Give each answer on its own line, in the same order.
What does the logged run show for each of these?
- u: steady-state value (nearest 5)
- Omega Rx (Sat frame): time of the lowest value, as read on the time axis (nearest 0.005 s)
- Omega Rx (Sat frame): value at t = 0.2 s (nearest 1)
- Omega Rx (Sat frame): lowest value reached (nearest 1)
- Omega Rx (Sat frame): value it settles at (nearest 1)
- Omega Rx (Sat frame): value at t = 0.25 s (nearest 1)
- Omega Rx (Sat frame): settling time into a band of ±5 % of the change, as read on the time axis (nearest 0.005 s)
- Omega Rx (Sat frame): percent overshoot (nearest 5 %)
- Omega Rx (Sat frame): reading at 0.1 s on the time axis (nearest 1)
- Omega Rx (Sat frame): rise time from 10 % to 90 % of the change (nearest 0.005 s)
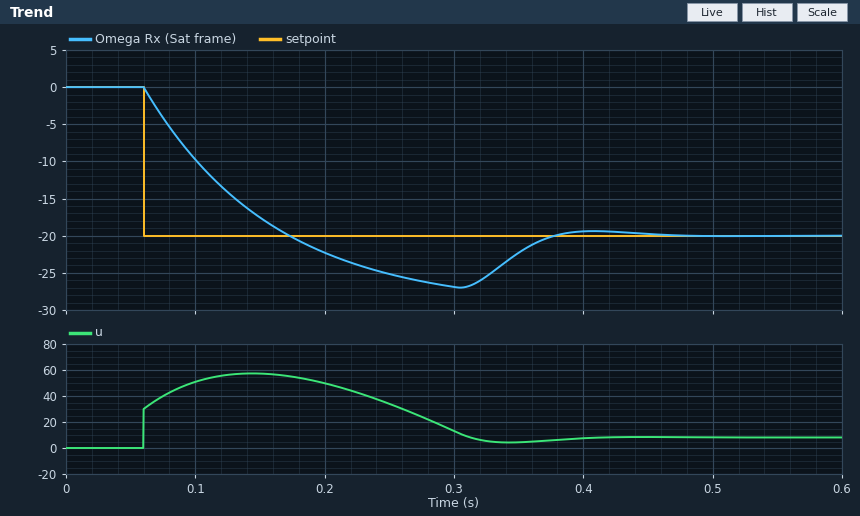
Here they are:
10
0.305 s
-22
-27
-20
-25
0.365 s
35 %
-10
0.085 s
